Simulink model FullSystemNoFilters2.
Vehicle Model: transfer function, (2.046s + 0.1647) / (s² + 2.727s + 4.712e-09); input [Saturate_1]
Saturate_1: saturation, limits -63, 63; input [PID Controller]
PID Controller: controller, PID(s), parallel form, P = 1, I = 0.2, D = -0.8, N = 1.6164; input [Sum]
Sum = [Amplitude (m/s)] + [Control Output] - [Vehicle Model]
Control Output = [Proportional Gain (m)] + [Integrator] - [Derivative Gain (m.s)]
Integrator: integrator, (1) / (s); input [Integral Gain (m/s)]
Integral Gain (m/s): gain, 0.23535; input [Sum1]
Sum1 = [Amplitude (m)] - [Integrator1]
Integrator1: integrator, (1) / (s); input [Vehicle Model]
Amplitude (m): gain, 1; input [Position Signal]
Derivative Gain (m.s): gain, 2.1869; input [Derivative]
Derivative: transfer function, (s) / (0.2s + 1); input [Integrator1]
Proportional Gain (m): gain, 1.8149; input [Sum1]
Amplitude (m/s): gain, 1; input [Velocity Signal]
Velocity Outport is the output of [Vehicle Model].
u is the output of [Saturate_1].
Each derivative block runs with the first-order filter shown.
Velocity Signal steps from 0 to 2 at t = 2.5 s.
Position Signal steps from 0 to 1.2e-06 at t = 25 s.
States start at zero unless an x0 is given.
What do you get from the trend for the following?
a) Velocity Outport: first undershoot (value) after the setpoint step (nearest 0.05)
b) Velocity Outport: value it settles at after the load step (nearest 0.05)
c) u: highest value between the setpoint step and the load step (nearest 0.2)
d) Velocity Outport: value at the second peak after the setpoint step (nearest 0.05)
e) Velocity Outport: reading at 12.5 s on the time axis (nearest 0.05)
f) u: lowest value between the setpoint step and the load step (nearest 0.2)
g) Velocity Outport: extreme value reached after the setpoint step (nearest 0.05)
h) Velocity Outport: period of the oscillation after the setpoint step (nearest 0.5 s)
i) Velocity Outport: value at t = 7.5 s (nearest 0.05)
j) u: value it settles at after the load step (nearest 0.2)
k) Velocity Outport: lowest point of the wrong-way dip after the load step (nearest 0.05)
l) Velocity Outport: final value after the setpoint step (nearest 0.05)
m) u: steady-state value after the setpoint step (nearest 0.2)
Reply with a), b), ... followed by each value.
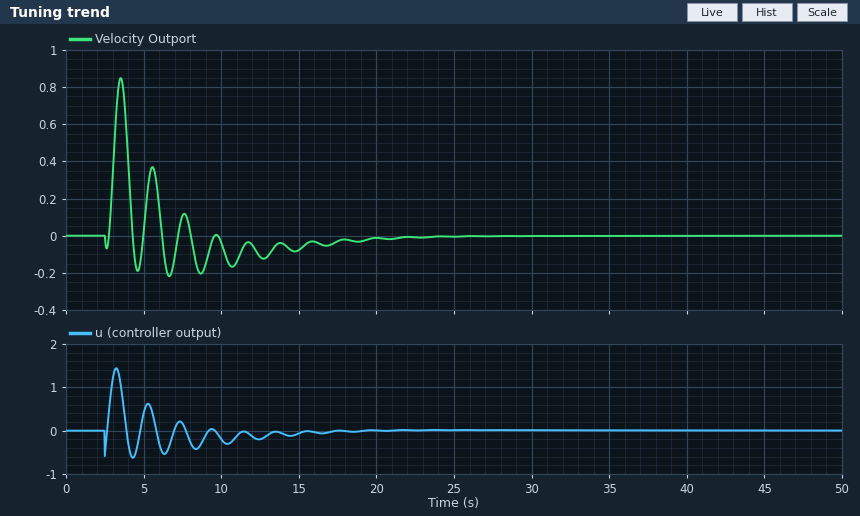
a) -0.20
b) 0.00
c) 1.4
d) 0.35
e) -0.10
f) -0.6
g) 0.85
h) 2.0 s
i) 0.10
j) 0.0
k) 0.00
l) 0.00
m) 0.0
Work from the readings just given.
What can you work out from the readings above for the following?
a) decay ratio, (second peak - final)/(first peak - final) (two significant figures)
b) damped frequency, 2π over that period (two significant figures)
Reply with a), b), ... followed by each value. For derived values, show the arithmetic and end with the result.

a) (0.35 - 0) / (0.85 - 0) = 0.41
b) 2π / 2 = 3.1 rad/s
